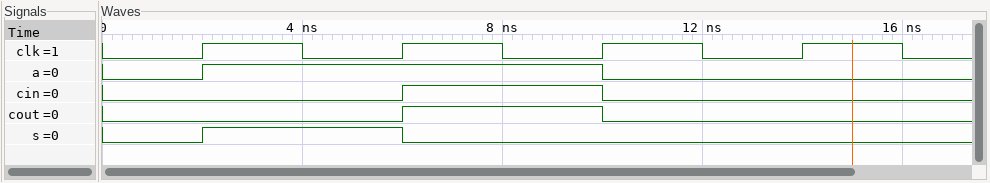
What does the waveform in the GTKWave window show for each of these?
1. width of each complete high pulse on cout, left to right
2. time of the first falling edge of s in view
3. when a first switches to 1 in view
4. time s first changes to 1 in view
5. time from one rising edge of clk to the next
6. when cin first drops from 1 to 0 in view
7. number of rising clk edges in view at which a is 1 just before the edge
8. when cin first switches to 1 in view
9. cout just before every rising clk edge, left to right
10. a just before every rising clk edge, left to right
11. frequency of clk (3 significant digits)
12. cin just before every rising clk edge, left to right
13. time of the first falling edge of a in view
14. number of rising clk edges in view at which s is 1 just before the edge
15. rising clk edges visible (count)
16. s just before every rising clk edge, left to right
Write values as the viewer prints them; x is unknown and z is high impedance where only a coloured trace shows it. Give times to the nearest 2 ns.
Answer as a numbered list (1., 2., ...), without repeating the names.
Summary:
1. 4 ns
2. 6 ns
3. 2 ns
4. 2 ns
5. 4 ns
6. 10 ns
7. 2
8. 6 ns
9. 0 0 1 0
10. 0 1 1 0
11. 250 MHz
12. 0 0 1 0
13. 10 ns
14. 1
15. 4
16. 0 1 0 0
